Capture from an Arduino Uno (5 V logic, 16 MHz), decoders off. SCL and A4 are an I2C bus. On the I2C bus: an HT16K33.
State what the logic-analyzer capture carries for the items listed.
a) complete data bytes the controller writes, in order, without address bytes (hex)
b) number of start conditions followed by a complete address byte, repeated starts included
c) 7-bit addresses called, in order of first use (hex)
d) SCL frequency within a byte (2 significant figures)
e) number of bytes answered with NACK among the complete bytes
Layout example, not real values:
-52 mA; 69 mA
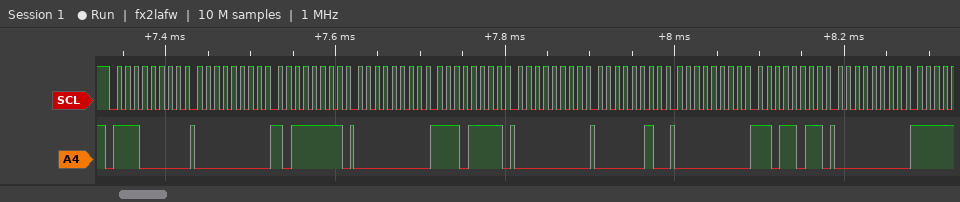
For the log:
00 BF 00 EF 00 02 00 DB 00; 1; 0x70; 100 kHz; 0
